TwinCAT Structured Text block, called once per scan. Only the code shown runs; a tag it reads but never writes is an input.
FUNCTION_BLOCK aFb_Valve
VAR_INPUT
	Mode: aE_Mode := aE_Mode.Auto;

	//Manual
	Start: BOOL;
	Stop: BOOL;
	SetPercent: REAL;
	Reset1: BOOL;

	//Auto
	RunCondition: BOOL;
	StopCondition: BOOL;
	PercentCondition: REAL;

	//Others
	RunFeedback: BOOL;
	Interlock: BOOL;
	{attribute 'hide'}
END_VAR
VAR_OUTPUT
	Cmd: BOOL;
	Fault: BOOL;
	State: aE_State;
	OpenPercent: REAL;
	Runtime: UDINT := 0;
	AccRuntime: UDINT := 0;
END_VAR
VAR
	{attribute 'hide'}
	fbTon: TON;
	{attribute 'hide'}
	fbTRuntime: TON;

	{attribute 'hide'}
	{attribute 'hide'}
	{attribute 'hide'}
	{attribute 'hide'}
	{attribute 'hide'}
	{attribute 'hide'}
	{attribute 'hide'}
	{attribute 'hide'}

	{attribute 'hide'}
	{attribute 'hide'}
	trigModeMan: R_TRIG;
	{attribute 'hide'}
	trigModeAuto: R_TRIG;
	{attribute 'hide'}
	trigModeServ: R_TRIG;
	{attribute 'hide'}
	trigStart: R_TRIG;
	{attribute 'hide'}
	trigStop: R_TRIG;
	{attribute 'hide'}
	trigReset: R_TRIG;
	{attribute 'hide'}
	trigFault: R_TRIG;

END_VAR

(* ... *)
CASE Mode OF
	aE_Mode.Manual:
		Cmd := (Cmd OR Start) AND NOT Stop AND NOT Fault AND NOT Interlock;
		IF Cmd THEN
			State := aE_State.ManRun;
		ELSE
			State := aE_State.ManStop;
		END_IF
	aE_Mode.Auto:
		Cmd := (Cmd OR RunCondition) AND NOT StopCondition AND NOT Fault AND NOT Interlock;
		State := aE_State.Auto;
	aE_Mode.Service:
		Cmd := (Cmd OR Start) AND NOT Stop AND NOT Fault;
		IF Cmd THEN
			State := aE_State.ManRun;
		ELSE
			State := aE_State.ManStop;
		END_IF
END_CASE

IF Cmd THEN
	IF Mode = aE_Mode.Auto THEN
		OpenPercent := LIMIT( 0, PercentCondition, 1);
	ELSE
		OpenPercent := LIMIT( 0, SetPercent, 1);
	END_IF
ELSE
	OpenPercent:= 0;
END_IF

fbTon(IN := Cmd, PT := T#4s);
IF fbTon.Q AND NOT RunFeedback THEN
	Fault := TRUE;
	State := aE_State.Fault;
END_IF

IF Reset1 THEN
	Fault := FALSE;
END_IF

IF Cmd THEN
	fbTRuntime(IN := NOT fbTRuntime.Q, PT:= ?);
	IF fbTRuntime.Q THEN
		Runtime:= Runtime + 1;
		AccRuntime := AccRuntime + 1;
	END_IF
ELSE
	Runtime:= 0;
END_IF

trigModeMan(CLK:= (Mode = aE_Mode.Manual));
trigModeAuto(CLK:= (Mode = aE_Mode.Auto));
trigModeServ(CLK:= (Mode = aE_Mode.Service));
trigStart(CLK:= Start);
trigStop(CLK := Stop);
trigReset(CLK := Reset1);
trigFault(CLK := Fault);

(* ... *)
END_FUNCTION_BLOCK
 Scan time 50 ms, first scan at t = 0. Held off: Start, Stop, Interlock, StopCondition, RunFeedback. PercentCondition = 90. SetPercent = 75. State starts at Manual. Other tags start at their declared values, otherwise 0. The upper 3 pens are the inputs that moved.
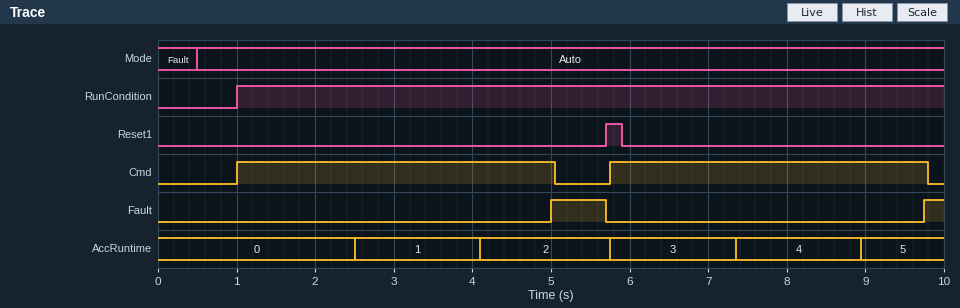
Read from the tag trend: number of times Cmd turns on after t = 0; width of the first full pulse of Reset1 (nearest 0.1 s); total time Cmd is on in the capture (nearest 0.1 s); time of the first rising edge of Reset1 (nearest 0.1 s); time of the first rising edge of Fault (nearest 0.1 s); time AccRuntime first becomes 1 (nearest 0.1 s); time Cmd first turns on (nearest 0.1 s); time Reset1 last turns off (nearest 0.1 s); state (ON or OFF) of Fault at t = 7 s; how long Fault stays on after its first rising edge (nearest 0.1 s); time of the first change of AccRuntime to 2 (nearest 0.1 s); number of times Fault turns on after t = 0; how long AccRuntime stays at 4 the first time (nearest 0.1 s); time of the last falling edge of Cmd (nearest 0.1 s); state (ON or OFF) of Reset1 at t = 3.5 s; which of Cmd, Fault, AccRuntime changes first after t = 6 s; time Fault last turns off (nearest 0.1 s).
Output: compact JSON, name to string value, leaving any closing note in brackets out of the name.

{"number of times Cmd turns on after t = 0": "2", "width of the first full pulse of Reset1": "0.2 s", "total time Cmd is on in the capture": "8.1 s", "time of the first rising edge of Reset1": "5.7 s", "time of the first rising edge of Fault": "5.0 s", "time AccRuntime first becomes 1": "2.5 s", "time Cmd first turns on": "1.0 s", "time Reset1 last turns off": "5.9 s", "state (ON or OFF) of Fault at t = 7 s": "OFF", "how long Fault stays on after its first rising edge": "0.7 s", "time of the first change of AccRuntime to 2": "4.1 s", "number of times Fault turns on after t = 0": "2", "how long AccRuntime stays at 4 the first time": "1.6 s", "time of the last falling edge of Cmd": "9.8 s", "state (ON or OFF) of Reset1 at t = 3.5 s": "OFF", "which of Cmd, Fault, AccRuntime changes first after t = 6 s": "AccRuntime", "time Fault last turns off": "5.7 s"}
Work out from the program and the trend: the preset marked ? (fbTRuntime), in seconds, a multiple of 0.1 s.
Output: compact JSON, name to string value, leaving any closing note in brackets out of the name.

{"the preset marked ? (fbTRuntime), in seconds, a multiple of 0.1 s": "1.5 s"}
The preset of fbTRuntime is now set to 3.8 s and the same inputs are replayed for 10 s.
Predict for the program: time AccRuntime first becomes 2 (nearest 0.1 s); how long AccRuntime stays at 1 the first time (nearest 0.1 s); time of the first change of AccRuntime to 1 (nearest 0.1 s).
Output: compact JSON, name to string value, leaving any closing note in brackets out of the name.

{"time AccRuntime first becomes 2": "8.7 s", "how long AccRuntime stays at 1 the first time": "3.9 s", "time of the first change of AccRuntime to 1": "4.8 s"}
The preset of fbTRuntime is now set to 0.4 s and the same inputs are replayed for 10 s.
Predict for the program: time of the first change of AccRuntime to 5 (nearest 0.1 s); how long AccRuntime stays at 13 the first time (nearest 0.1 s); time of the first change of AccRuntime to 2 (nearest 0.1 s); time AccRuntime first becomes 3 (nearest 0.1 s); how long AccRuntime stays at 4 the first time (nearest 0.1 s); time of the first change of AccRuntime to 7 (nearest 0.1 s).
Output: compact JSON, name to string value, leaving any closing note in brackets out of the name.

{"time of the first change of AccRuntime to 5": "3.4 s", "how long AccRuntime stays at 13 the first time": "0.5 s", "time of the first change of AccRuntime to 2": "1.9 s", "time AccRuntime first becomes 3": "2.4 s", "how long AccRuntime stays at 4 the first time": "0.5 s", "time of the first change of AccRuntime to 7": "4.4 s"}
